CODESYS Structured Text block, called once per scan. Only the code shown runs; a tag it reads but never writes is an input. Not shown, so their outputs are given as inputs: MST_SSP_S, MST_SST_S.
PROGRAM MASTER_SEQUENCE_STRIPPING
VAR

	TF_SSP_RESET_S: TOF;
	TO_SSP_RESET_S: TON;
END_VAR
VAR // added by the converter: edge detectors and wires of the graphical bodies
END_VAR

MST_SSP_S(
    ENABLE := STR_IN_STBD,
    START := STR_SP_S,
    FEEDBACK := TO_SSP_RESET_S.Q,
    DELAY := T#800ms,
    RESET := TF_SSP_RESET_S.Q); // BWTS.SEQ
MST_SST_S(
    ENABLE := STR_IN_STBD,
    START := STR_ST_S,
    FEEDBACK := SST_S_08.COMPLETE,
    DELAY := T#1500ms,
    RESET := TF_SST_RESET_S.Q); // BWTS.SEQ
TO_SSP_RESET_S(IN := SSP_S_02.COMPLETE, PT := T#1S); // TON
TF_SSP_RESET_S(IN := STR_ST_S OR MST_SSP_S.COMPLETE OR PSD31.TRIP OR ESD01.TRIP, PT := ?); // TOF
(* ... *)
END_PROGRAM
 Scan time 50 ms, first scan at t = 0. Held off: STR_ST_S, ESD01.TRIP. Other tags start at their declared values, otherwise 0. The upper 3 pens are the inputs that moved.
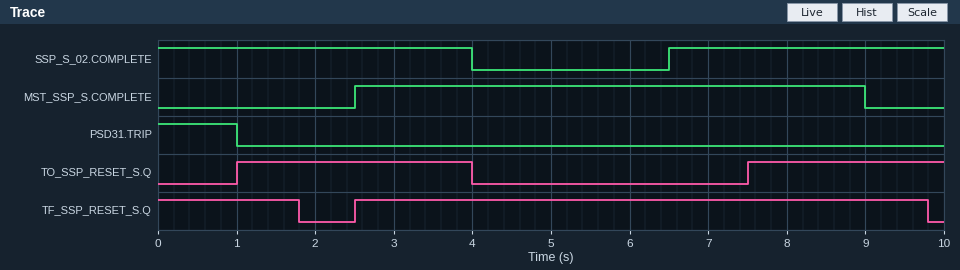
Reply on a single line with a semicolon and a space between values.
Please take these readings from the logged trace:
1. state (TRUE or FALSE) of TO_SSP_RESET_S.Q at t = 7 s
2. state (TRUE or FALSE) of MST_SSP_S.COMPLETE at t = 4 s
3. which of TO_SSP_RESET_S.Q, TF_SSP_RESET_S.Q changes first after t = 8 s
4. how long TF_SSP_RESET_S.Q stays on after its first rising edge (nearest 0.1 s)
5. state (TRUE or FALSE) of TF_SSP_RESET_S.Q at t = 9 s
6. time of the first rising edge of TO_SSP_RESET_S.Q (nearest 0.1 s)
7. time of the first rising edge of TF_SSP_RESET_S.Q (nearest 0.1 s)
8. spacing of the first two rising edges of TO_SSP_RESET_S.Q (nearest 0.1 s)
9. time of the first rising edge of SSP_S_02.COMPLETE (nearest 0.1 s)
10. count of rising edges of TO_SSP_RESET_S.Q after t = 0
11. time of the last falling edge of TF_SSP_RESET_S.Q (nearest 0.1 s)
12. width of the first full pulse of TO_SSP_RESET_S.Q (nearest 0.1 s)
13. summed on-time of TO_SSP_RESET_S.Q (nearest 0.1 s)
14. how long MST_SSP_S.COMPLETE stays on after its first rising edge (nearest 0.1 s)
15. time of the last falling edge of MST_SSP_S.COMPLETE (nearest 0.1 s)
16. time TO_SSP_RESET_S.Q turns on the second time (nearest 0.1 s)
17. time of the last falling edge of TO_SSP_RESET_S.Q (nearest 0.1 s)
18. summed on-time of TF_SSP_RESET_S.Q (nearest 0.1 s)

FALSE; TRUE; TF_SSP_RESET_S.Q; 7.3 s; TRUE; 1.0 s; 2.5 s; 6.5 s; 6.5 s; 2; 9.8 s; 3.0 s; 5.5 s; 6.5 s; 9.0 s; 7.5 s; 4.0 s; 9.1 s
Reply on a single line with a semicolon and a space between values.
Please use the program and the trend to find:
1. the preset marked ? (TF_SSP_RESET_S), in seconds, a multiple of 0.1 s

0.8 s
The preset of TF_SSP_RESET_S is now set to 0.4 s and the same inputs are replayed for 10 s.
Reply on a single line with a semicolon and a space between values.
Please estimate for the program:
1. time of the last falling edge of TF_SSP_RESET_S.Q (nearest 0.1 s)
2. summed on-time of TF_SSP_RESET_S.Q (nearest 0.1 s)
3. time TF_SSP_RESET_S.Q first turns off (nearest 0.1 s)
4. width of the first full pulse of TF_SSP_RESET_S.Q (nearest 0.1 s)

9.4 s; 8.3 s; 1.4 s; 6.9 s
